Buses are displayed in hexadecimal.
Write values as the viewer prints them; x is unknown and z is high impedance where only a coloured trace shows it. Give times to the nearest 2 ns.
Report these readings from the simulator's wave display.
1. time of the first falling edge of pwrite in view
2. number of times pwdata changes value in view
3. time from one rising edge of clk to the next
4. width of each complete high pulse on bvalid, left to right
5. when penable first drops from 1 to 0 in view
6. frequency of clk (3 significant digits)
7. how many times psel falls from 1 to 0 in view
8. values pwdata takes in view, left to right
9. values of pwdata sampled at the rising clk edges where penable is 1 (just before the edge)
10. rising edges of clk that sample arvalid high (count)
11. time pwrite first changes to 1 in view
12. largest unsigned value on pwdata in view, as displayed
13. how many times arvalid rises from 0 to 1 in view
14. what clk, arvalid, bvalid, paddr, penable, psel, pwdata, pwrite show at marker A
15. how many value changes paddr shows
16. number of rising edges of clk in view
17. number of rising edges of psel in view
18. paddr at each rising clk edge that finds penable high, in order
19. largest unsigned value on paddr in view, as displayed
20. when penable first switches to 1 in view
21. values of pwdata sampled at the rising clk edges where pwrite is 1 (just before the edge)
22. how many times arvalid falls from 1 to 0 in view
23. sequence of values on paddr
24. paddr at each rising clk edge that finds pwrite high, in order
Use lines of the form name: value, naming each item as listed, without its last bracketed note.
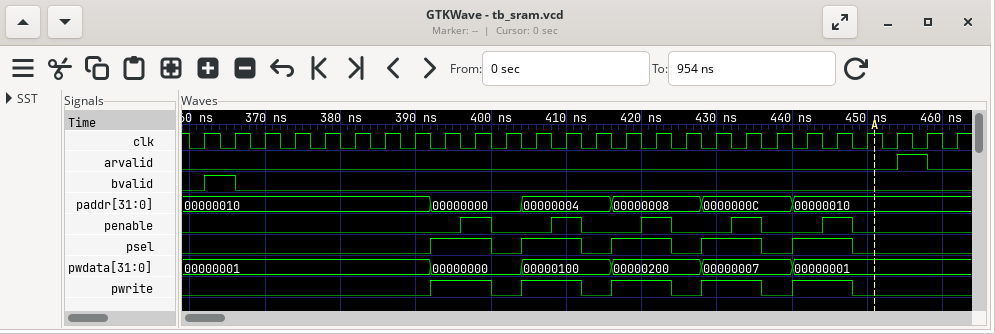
time of the first falling edge of pwrite in view: 400 ns
number of times pwdata changes value in view: 5
time from one rising edge of clk to the next: 4 ns
width of each complete high pulse on bvalid, left to right: 4 ns
when penable first drops from 1 to 0 in view: 400 ns
frequency of clk: 250 MHz
how many times psel falls from 1 to 0 in view: 5
values pwdata takes in view, left to right: 00000001, 00000000, 00000100, 00000200, 00000007, 00000001
values of pwdata sampled at the rising clk edges where penable is 1: 00000000, 00000100, 00000200, 00000007, 00000001
rising edges of clk that sample arvalid high: 1
time pwrite first changes to 1 in view: 392 ns
largest unsigned value on pwdata in view, as displayed: 00000200
how many times arvalid rises from 0 to 1 in view: 1
what clk, arvalid, bvalid, paddr, penable, psel, pwdata, pwrite show at marker A: clk=1, arvalid=0, bvalid=0, paddr=00000010, penable=0, psel=0, pwdata=00000001, pwrite=0
how many value changes paddr shows: 5
number of rising edges of clk in view: 26
number of rising edges of psel in view: 5
paddr at each rising clk edge that finds penable high, in order: 00000000, 00000004, 00000008, 0000000C, 00000010
largest unsigned value on paddr in view, as displayed: 00000010
when penable first switches to 1 in view: 396 ns
values of pwdata sampled at the rising clk edges where pwrite is 1: 00000000, 00000000, 00000100, 00000100, 00000200, 00000200, 00000007, 00000007, 00000001, 00000001
how many times arvalid falls from 1 to 0 in view: 1
sequence of values on paddr: 00000010, 00000000, 00000004, 00000008, 0000000C, 00000010
paddr at each rising clk edge that finds pwrite high, in order: 00000000, 00000000, 00000004, 00000004, 00000008, 00000008, 0000000C, 0000000C, 00000010, 00000010
